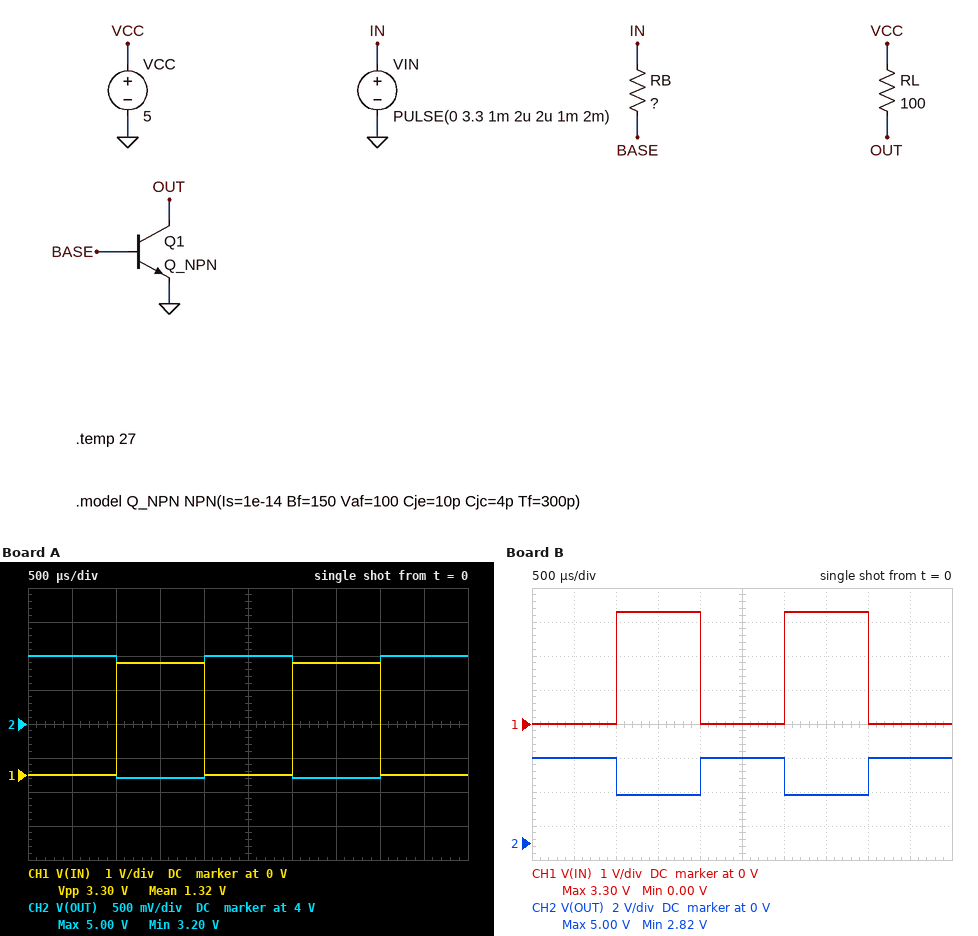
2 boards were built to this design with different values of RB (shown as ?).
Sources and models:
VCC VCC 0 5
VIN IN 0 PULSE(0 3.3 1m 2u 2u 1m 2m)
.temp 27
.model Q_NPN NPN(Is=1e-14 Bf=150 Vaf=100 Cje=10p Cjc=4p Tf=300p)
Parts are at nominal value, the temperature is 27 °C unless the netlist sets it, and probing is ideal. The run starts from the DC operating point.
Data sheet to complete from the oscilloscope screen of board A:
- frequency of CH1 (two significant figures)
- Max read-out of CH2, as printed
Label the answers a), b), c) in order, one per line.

a) 500 Hz
b) 5.00 V
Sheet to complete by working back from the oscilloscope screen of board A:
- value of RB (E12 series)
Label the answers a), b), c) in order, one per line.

a) 22 kΩ
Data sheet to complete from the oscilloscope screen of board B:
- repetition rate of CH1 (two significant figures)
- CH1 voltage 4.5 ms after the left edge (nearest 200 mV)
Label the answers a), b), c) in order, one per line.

a) 500 Hz
b) 0 V
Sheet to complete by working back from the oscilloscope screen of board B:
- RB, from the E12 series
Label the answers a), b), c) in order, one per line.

a) 18 kΩ
